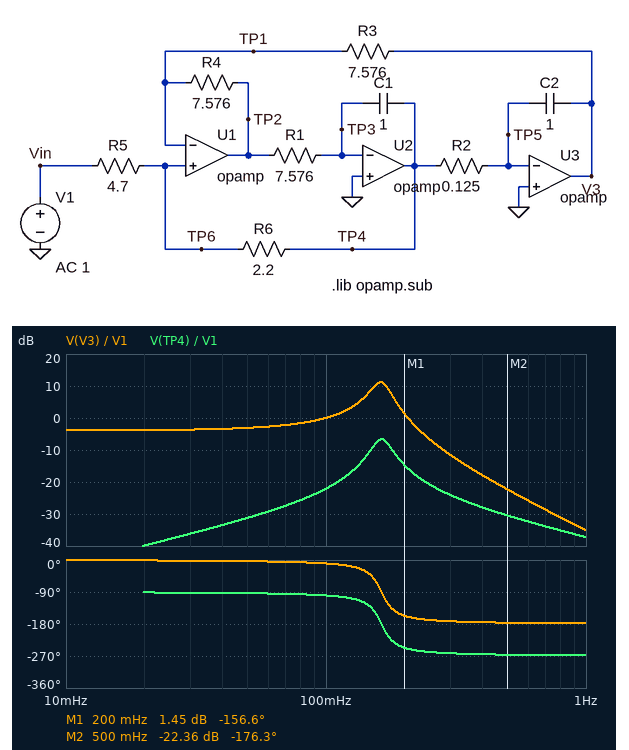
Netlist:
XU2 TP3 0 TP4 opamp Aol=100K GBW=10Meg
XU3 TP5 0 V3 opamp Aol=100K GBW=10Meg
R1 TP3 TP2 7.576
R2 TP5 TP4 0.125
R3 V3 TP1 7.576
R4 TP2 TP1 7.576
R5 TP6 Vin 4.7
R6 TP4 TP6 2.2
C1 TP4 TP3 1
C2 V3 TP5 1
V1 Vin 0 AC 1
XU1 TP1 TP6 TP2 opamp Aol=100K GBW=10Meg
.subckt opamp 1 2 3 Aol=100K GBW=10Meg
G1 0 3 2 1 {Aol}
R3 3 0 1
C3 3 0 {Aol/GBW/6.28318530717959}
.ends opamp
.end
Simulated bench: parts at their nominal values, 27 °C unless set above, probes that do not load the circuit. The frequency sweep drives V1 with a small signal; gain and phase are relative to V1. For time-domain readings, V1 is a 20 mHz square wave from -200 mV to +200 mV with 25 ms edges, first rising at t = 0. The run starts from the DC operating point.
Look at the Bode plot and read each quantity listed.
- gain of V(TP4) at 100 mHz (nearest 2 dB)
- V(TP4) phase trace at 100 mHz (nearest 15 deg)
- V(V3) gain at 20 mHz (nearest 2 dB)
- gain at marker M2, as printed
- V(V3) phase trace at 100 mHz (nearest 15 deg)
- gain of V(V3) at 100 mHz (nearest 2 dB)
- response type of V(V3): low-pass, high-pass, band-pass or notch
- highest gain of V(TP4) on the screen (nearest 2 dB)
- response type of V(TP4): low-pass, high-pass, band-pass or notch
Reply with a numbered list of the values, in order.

1. -22 dB
2. -105 deg
3. -4 dB
4. -22.36 dB
5. -15 deg
6. 0 dB
7. low-pass
8. -6 dB
9. band-pass
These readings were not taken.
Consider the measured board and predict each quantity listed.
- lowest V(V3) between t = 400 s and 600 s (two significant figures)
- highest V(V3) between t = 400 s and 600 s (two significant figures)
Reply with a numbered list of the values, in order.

1. -300 mV
2. 300 mV
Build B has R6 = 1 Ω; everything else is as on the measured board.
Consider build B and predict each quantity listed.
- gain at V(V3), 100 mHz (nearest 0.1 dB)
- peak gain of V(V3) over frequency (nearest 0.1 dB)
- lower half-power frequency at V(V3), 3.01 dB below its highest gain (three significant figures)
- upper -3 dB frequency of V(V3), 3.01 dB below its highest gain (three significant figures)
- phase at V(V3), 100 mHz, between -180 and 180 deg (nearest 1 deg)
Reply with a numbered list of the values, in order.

1. -5.2 dB
2. 4.4 dB
3. 143 mHz
4. 178 mHz
5. -12 deg
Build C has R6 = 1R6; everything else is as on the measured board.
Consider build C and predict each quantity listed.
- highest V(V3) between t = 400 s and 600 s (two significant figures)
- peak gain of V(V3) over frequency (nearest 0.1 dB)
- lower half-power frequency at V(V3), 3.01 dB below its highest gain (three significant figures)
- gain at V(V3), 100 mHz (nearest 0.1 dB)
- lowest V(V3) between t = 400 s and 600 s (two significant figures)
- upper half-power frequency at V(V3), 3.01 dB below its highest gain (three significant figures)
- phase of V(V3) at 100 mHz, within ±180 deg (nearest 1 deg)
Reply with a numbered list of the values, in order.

1. 240 mV
2. 8.5 dB
3. 145 mHz
4. -2.0 dB
5. -240 mV
6. 177 mHz
7. -11 deg
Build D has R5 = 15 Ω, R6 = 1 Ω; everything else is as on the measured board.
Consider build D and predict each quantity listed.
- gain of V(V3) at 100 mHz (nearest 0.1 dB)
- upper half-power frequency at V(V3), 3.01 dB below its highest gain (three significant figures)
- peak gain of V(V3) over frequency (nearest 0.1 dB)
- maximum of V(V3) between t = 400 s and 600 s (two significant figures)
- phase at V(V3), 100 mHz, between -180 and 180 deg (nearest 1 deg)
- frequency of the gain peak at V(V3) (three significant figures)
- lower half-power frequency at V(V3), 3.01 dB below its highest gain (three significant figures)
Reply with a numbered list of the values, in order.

1. -14.2 dB
2. 180 mHz
3. -5.6 dB
4. 58 mV
5. -13 deg
6. 161 mHz
7. 140 mHz
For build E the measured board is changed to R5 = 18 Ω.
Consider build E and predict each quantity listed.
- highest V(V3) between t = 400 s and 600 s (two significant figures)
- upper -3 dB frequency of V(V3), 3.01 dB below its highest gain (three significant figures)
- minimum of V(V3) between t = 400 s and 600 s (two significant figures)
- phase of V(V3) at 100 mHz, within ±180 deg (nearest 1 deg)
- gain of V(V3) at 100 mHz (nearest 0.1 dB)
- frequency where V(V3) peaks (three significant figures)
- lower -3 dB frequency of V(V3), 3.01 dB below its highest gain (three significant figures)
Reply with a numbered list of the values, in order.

1. 100 mV
2. 179 mHz
3. -100 mV
4. -13 deg
5. -9.4 dB
6. 161 mHz
7. 141 mHz
